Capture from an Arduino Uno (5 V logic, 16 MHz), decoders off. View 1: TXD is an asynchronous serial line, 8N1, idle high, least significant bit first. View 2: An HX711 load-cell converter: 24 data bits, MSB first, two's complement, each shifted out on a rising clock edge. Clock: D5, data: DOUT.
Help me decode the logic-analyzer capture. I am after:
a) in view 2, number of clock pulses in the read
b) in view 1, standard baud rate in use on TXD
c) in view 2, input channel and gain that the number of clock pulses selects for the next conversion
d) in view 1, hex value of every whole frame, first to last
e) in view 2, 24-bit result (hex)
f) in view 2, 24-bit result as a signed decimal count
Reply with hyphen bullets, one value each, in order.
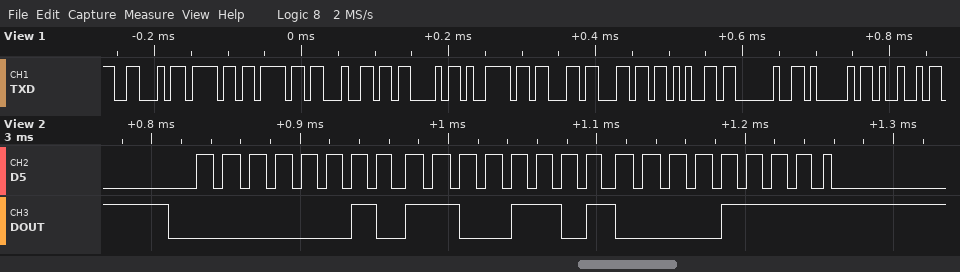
- 25
- 115200 baud
- channel A, gain 128
- 46 6F 6F 64 43 79 63 6C 65 20 41 49
- 0x02CD0F
- 183567
